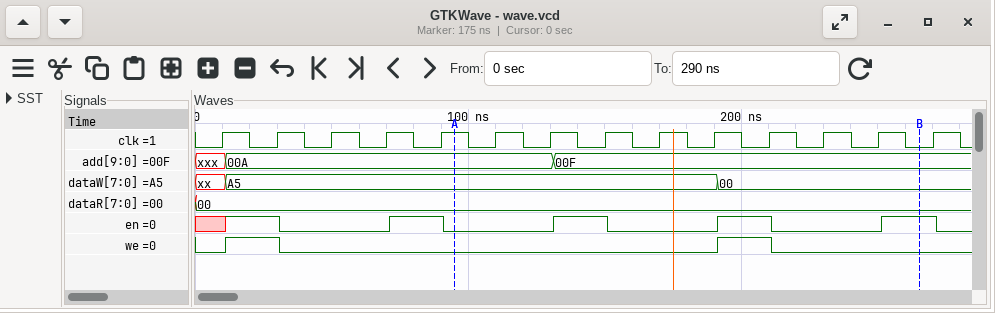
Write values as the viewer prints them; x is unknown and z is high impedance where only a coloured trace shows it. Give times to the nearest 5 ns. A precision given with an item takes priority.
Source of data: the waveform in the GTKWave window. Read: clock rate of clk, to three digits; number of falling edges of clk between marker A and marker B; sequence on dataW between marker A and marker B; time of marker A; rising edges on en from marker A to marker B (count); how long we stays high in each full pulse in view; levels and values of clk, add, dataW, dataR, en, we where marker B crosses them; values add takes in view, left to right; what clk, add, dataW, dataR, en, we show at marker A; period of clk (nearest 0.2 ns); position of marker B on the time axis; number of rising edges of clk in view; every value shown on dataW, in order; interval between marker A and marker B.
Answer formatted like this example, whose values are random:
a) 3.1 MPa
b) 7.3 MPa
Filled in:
a) 50.0 MHz
b) 9
c) A5, 00
d) 95 ns
e) 3
f) 20 ns, 20 ns
g) clk=0, add=00F, dataW=00, dataR=00, en=1, we=0
h) xxx, 00A, 00F
i) clk=1, add=00A, dataW=A5, dataR=00, en=0, we=0
j) 20 ns
k) 265 ns
l) 14
m) xx, A5, 00
n) 170 ns
